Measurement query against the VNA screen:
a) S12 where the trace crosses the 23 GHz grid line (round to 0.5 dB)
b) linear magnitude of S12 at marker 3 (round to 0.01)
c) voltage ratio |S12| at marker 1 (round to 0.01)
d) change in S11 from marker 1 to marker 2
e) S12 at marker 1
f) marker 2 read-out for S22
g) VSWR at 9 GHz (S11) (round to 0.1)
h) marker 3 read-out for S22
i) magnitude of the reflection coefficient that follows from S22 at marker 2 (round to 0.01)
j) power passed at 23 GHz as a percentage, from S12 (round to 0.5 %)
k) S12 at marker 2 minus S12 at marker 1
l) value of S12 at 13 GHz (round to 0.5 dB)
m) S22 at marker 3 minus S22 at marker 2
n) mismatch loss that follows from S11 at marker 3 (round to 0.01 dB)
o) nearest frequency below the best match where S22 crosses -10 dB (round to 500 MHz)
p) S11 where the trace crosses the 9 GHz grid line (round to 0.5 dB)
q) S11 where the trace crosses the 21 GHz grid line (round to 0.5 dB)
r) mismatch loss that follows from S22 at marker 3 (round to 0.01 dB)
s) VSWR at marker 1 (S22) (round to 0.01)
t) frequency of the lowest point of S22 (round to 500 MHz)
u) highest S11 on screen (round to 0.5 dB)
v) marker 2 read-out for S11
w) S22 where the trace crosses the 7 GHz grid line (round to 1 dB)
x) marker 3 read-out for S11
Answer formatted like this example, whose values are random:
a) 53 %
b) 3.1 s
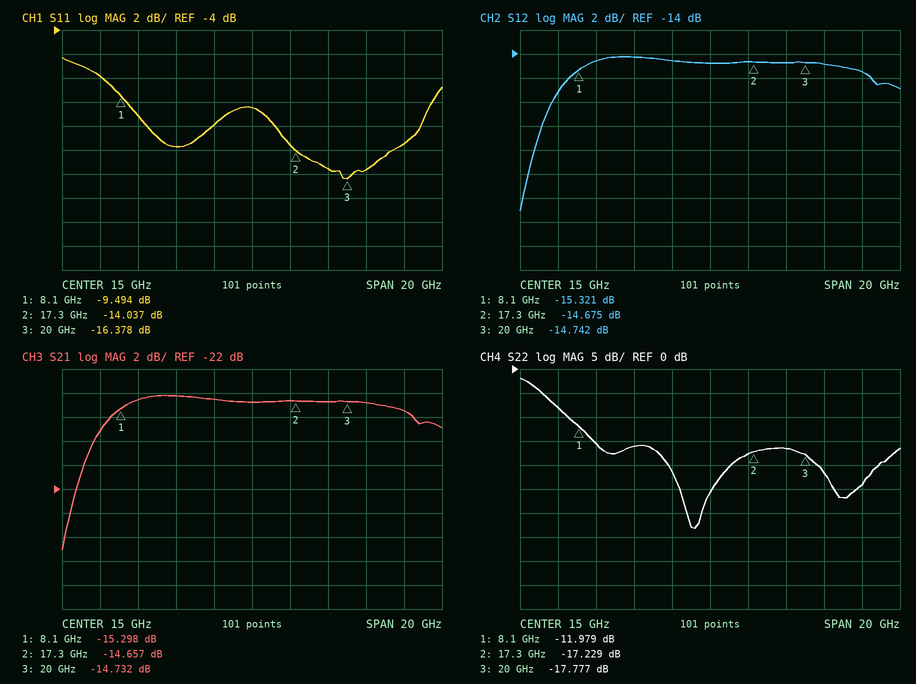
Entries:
a) -15.5 dB
b) 0.18
c) 0.17
d) -4.543 dB
e) -15.321 dB
f) -17.229 dB
g) 1.8
h) -17.777 dB
i) 0.14
j) 3.0 %
k) 0.646 dB
l) -14.5 dB
m) -0.548 dB
n) 0.10 dB
o) 7.5 GHz
p) -11.0 dB
q) -15.5 dB
r) 0.07 dB
s) 1.67
t) 14.0 GHz
u) -6.5 dB
v) -14.037 dB
w) -8 dB
x) -16.378 dB
